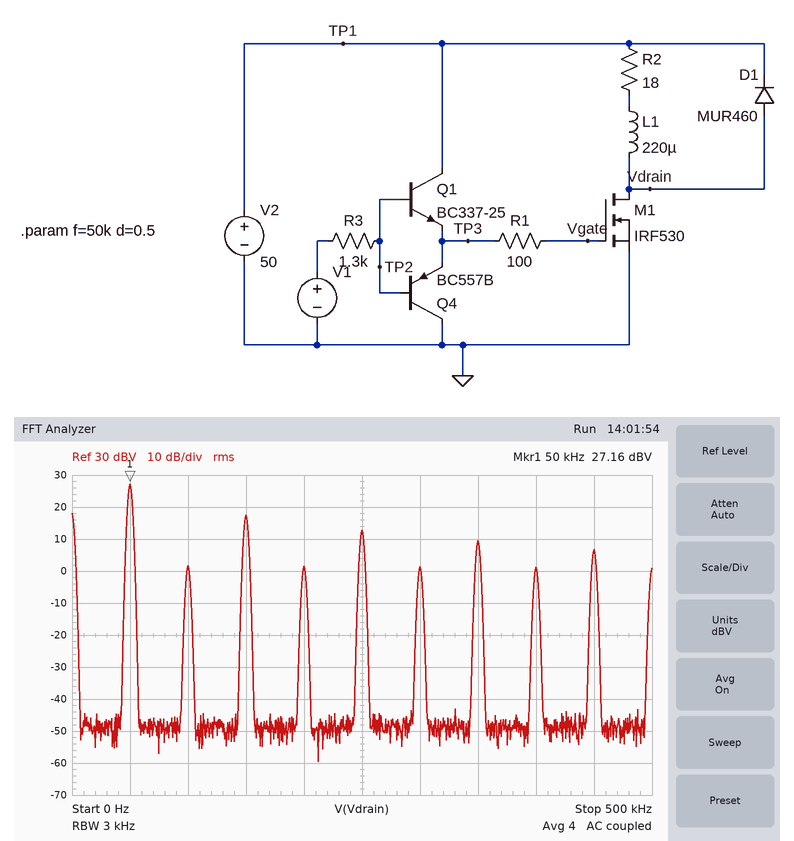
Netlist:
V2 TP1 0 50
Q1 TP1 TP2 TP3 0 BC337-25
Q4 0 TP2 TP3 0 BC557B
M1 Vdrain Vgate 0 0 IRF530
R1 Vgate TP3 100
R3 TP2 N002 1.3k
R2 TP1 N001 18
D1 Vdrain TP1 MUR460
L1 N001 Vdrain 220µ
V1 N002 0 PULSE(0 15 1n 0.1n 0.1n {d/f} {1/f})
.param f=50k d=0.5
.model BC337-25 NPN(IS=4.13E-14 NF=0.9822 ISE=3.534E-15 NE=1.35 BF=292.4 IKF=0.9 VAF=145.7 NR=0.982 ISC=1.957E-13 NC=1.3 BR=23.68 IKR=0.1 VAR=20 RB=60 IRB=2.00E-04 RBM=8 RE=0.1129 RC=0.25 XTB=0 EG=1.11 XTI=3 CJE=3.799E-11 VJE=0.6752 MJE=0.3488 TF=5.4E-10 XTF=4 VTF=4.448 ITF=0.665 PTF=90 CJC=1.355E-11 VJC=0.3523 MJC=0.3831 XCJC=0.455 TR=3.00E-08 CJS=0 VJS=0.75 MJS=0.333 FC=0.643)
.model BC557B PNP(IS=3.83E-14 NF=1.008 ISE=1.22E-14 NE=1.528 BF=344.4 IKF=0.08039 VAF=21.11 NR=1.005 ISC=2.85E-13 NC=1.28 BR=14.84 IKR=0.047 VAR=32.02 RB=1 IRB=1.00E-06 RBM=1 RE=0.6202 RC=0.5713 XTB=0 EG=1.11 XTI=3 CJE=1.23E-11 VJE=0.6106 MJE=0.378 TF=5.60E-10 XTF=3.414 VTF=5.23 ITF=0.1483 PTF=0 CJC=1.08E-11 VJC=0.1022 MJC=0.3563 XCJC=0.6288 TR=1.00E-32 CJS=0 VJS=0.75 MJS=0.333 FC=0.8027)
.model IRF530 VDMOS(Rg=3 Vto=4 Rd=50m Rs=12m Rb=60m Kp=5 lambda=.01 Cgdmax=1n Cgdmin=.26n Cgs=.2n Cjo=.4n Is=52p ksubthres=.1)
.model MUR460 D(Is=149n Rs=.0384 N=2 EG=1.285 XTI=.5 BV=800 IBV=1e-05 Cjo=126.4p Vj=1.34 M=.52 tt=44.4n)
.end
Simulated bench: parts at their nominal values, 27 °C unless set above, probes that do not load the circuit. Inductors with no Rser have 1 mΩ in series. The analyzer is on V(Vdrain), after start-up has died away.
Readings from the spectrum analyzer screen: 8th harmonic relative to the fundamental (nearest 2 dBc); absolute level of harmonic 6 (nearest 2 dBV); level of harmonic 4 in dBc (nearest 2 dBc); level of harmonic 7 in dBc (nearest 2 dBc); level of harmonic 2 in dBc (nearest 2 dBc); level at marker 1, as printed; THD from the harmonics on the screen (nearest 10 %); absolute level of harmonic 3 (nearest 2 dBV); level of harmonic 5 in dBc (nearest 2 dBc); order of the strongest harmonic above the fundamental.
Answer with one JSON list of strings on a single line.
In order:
["-26 dBc", "2 dBV", "-26 dBc", "-18 dBc", "-26 dBc", "27.16 dBV", "40 %", "18 dBV", "-14 dBc", "3"]
